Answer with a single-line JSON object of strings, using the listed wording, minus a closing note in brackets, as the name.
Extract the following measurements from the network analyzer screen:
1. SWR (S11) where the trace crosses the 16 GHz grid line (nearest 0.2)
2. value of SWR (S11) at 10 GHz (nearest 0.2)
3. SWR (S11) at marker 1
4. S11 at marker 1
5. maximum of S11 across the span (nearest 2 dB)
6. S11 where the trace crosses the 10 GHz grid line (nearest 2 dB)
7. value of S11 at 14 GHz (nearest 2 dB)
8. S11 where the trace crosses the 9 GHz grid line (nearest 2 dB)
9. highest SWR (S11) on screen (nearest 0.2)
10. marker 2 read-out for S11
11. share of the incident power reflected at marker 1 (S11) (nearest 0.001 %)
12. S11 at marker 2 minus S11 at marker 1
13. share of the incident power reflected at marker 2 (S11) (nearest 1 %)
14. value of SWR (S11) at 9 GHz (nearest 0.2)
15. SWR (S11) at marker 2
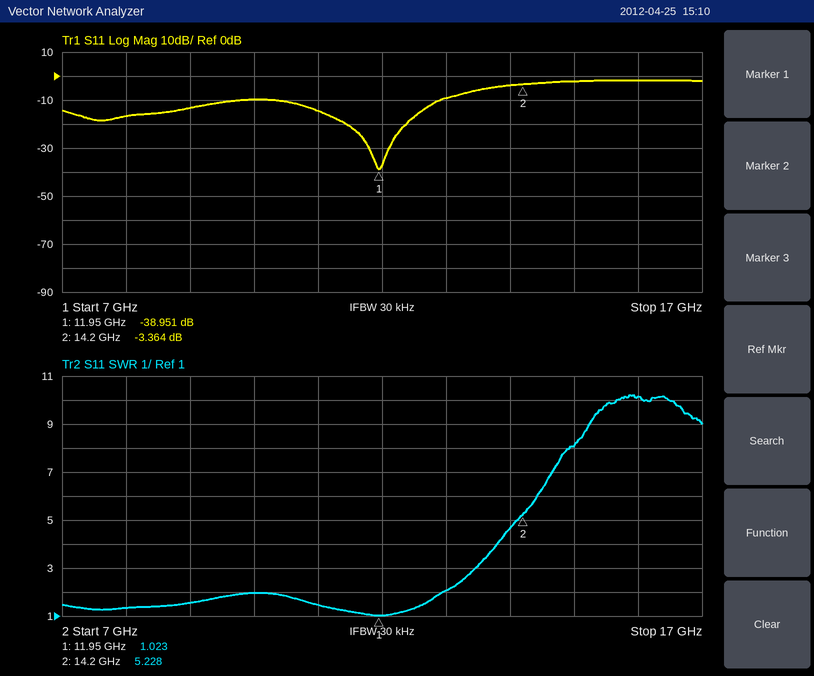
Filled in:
{"SWR (S11) where the trace crosses the 16 GHz grid line": "10.2", "value of SWR (S11) at 10 GHz": "2.0", "SWR (S11) at marker 1": "1.023", "S11 at marker 1": "-38.951 dB", "maximum of S11 across the span": "-2 dB", "S11 where the trace crosses the 10 GHz grid line": "-10 dB", "value of S11 at 14 GHz": "-4 dB", "S11 where the trace crosses the 9 GHz grid line": "-14 dB", "highest SWR (S11) on screen": "10.2", "marker 2 read-out for S11": "-3.364 dB", "share of the incident power reflected at marker 1 (S11)": "0.013 %", "S11 at marker 2 minus S11 at marker 1": "35.587 dB", "share of the incident power reflected at marker 2 (S11)": "46 %", "value of SWR (S11) at 9 GHz": "1.6", "SWR (S11) at marker 2": "5.228"}
